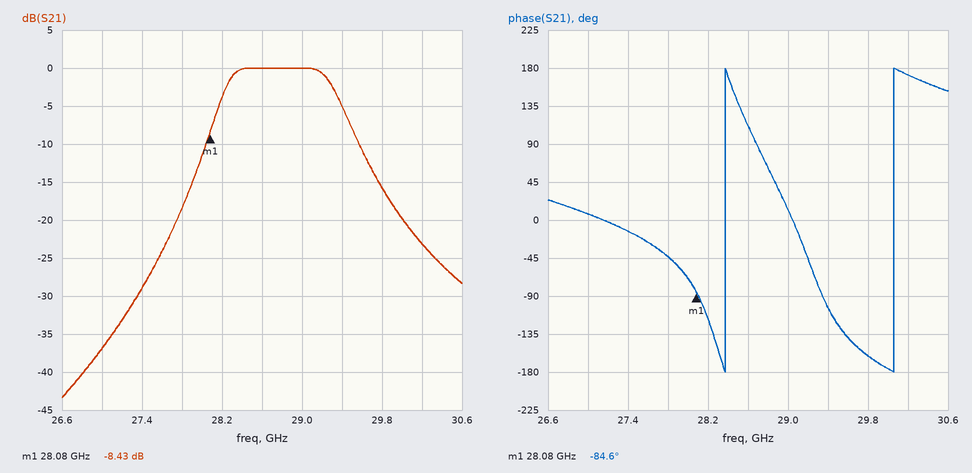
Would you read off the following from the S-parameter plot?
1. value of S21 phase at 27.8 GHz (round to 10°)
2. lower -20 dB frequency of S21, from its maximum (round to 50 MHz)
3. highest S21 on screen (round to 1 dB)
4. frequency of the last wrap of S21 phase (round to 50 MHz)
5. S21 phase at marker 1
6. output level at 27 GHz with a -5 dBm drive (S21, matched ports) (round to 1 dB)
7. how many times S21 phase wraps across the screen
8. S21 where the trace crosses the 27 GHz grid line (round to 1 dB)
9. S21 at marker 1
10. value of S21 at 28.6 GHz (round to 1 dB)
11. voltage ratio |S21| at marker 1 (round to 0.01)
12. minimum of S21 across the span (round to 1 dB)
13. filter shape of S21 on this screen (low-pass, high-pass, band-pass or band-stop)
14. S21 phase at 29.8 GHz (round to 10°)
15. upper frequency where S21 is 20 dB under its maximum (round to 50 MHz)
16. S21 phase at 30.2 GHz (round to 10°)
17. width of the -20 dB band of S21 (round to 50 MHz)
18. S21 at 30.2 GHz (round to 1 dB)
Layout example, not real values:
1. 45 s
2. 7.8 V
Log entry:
1. -40°
2. 27.75 GHz
3. 0 dB
4. 30.05 GHz
5. -84.6°
6. -42 dBm
7. 2
8. -37 dB
9. -8.43 dB
10. 0 dB
11. 0.38
12. -43 dB
13. band-pass
14. -160°
15. 30.00 GHz
16. 170°
17. 2.25 GHz
18. -23 dB
